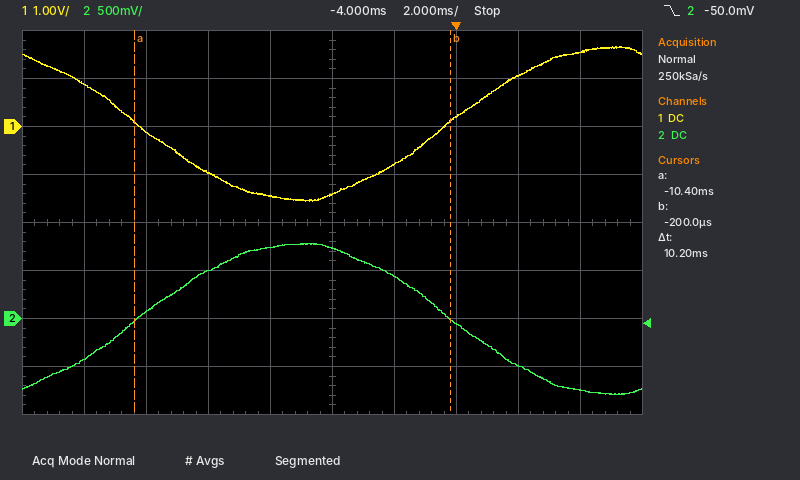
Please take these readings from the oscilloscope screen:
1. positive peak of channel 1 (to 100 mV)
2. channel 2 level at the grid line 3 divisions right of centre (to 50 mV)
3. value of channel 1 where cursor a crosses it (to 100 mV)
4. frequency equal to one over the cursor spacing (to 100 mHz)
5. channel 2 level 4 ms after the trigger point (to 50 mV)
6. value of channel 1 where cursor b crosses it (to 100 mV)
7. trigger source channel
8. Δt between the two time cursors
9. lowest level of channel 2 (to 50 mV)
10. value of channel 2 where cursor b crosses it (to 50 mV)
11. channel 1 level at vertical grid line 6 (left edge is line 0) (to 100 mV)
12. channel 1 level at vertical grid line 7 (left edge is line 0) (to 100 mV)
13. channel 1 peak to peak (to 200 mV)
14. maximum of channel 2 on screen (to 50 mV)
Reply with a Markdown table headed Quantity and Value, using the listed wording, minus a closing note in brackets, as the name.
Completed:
| Quantity | Value |
|---|---|
| positive peak of channel 1 | 1.7 V |
| channel 2 level at the grid line 3 divisions right of centre | -500 mV |
| value of channel 1 where cursor a crosses it | 100 mV |
| frequency equal to one over the cursor spacing | 98.0 Hz |
| channel 2 level 4 ms after the trigger point | -750 mV |
| value of channel 1 where cursor b crosses it | 100 mV |
| trigger source channel | channel 2 |
| Δt between the two time cursors | 10.2 ms |
| lowest level of channel 2 | -800 mV |
| value of channel 2 where cursor b crosses it | 0 mV |
| channel 1 level at vertical grid line 6 (left edge is line 0) | -800 mV |
| channel 1 level at vertical grid line 7 (left edge is line 0) | 200 mV |
| channel 1 peak to peak | 3.2 V |
| maximum of channel 2 on screen | 800 mV |
